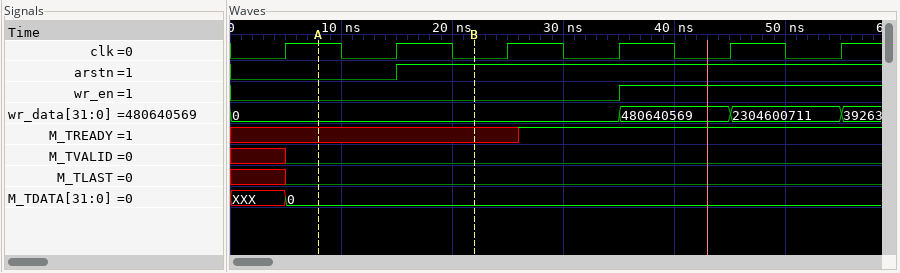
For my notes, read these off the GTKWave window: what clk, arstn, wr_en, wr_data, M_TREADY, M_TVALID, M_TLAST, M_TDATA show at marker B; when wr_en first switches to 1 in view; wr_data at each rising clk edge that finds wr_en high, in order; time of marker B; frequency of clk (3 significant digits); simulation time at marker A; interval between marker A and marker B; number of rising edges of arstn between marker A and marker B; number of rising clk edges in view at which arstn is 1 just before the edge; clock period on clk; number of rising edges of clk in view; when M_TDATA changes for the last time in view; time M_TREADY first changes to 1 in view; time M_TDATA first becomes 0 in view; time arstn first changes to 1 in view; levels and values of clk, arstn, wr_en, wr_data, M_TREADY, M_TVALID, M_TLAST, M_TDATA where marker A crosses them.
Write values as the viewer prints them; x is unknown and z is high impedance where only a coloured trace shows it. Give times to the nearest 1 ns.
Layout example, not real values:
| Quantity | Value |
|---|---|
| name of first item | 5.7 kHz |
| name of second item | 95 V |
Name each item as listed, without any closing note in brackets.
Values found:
| Quantity | Value |
|---|---|
| what clk, arstn, wr_en, wr_data, M_TREADY, M_TVALID, M_TLAST, M_TDATA show at marker B | clk=0, arstn=1, wr_en=0, wr_data=0, M_TREADY=x, M_TVALID=0, M_TLAST=0, M_TDATA=0 |
| when wr_en first switches to 1 in view | 35 ns |
| wr_data at each rising clk edge that finds wr_en high, in order | 480640569, 2304600711 |
| time of marker B | 22 ns |
| frequency of clk | 100 MHz |
| simulation time at marker A | 8 ns |
| interval between marker A and marker B | 14 ns |
| number of rising edges of arstn between marker A and marker B | 1 |
| number of rising clk edges in view at which arstn is 1 just before the edge | 4 |
| clock period on clk | 10 ns |
| number of rising edges of clk in view | 6 |
| when M_TDATA changes for the last time in view | 5 ns |
| time M_TREADY first changes to 1 in view | 26 ns |
| time M_TDATA first becomes 0 in view | 5 ns |
| time arstn first changes to 1 in view | 15 ns |
| levels and values of clk, arstn, wr_en, wr_data, M_TREADY, M_TVALID, M_TLAST, M_TDATA where marker A crosses them | clk=1, arstn=0, wr_en=0, wr_data=0, M_TREADY=x, M_TVALID=0, M_TLAST=0, M_TDATA=0 |
